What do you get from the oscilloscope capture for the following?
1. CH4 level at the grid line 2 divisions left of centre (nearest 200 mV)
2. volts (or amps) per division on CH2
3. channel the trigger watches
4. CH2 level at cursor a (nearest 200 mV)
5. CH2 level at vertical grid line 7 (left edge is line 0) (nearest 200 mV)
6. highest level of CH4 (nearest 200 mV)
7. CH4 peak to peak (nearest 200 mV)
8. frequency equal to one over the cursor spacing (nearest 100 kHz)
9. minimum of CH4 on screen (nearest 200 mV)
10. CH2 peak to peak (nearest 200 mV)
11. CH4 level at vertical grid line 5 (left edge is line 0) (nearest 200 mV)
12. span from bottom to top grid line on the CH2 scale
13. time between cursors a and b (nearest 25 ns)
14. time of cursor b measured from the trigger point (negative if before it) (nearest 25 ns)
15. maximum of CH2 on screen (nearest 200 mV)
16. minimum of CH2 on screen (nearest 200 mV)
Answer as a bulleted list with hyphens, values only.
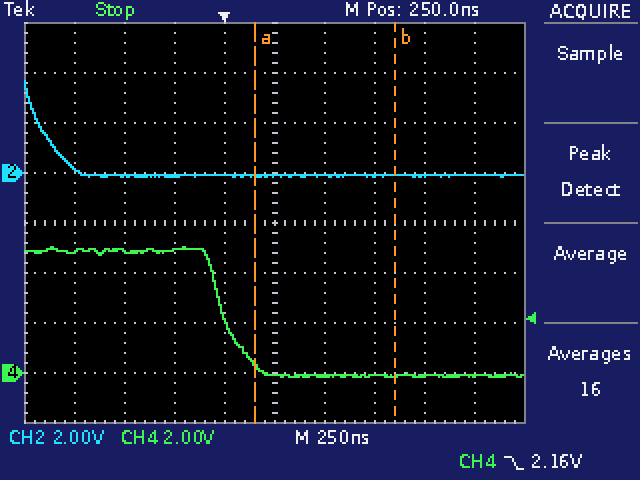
- 5.0 V
- 2 V
- CH4
- -200 mV
- -200 mV
- 5.0 V
- 5.2 V
- 1.4 MHz
- -200 mV
- 3.8 V
- 0.0 V
- 16 V
- 700 ns
- +850 ns
- 3.6 V
- -200 mV
